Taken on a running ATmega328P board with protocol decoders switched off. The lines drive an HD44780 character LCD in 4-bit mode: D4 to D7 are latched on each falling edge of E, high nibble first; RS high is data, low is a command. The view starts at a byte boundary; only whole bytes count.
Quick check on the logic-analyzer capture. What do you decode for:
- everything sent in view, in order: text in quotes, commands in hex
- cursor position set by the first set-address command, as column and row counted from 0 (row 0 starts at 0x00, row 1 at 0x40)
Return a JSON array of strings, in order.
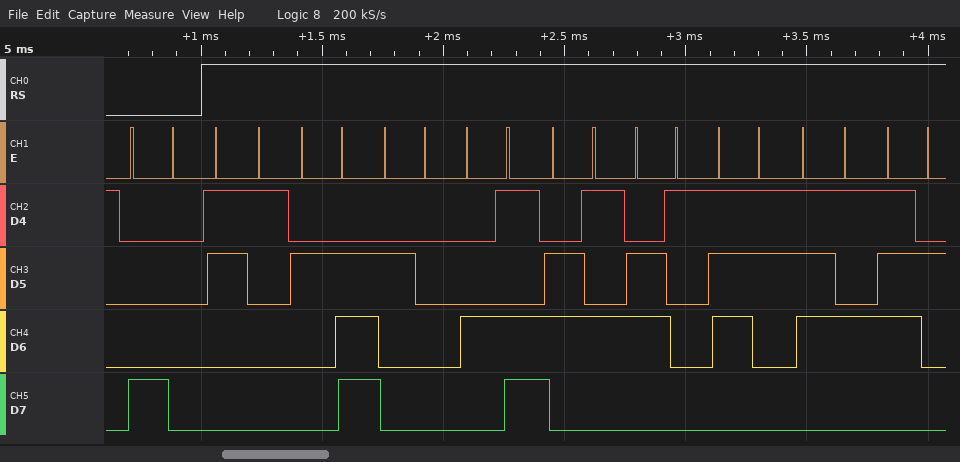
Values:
["0x80 \"1. Measur\"", "column 0, row 0"]
